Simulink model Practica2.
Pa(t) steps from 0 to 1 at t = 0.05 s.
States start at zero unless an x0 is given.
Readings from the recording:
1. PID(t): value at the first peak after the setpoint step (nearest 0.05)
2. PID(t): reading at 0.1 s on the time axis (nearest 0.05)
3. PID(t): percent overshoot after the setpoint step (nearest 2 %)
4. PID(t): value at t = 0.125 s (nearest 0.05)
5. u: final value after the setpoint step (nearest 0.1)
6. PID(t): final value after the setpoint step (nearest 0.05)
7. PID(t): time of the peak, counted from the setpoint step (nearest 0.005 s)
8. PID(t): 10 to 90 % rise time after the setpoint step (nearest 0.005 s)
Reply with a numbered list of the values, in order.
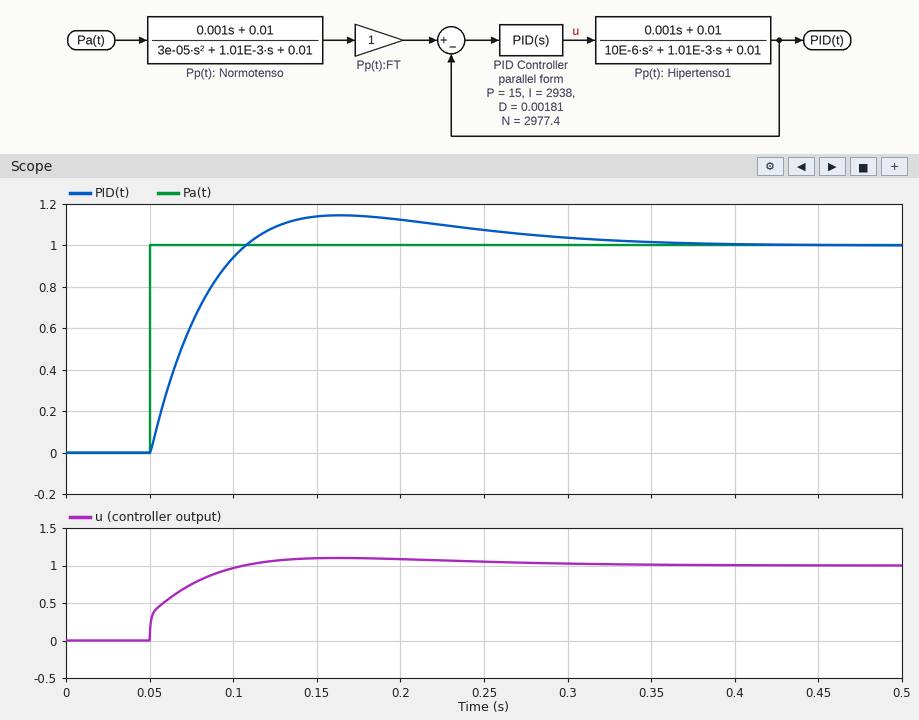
1. 1.15
2. 0.95
3. 14 %
4. 1.10
5. 1.0
6. 1.00
7. 0.115 s
8. 0.040 s
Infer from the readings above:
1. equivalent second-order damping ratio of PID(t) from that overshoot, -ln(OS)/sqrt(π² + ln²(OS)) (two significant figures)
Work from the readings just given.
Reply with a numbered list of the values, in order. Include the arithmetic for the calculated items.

1. ln(0.14) = -1.966; 1.966 / sqrt(9.870 + 3.866) = 0.53
